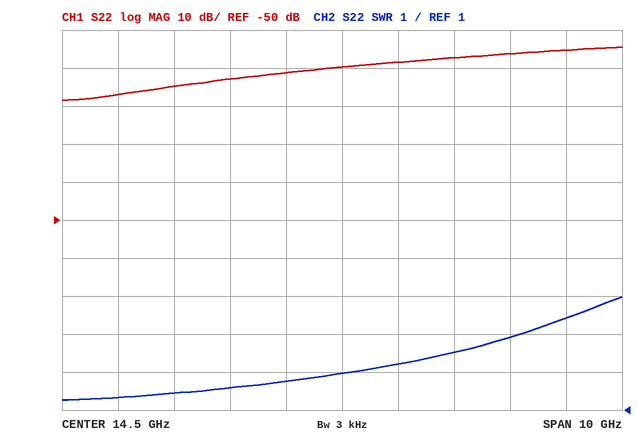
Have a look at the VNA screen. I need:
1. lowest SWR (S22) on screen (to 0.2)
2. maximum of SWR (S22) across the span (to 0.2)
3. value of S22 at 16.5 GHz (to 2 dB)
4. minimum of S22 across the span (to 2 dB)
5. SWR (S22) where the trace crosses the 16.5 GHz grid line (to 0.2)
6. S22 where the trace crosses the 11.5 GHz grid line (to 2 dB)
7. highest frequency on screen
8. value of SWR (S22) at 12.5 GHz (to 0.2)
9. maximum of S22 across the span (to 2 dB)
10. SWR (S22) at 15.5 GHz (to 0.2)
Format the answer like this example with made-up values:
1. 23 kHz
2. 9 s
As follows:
1. 1.2
2. 4.0
3. -8 dB
4. -18 dB
5. 2.6
6. -14 dB
7. 19.5 GHz
8. 1.6
9. -4 dB
10. 2.2
